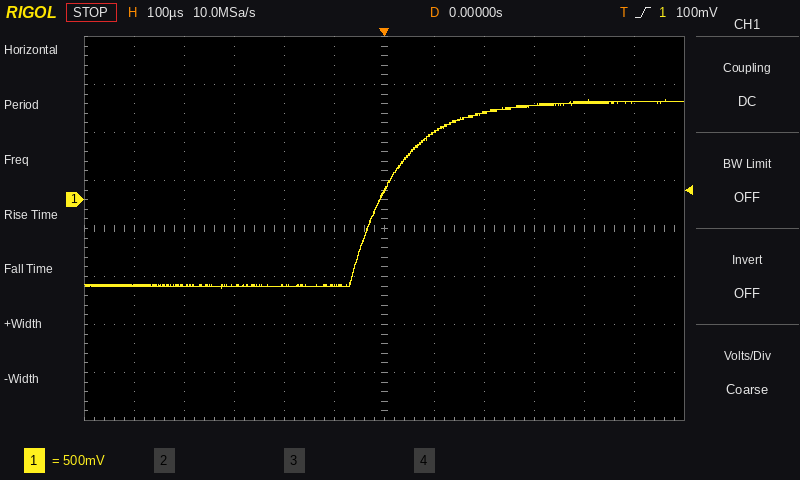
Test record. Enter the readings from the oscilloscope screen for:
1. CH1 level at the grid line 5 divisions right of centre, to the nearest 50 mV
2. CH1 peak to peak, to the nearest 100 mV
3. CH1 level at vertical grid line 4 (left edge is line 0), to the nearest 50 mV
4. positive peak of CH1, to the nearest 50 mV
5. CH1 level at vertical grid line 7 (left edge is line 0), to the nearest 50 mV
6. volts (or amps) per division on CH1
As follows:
1.00 V
2.00 V
-900 mV
1.05 V
700 mV
500 mV
